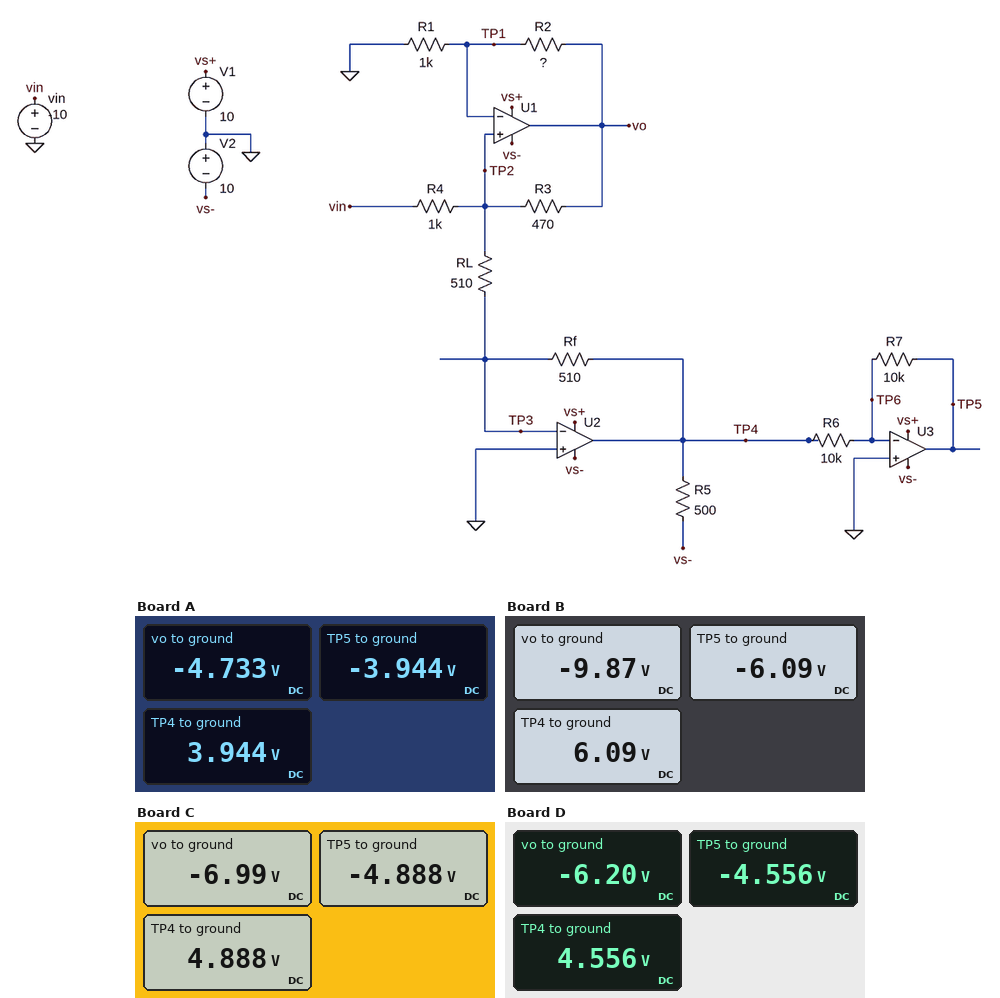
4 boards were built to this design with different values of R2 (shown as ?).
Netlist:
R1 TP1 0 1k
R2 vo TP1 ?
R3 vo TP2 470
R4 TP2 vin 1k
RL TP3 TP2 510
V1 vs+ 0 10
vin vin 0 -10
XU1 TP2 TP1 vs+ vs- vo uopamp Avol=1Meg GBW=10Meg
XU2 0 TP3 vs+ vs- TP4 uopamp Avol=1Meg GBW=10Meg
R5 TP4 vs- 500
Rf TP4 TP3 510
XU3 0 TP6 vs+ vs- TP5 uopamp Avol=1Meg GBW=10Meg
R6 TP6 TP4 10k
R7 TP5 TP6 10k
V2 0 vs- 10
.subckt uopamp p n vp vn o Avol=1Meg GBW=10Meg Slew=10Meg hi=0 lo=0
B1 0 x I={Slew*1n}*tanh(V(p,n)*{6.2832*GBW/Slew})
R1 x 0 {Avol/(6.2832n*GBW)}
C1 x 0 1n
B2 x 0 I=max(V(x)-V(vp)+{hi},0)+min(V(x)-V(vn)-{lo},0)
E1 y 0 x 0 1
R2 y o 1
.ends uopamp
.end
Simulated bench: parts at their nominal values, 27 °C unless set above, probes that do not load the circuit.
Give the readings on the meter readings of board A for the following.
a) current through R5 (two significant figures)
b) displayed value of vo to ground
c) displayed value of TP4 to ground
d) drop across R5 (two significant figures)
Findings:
28 mA
-4.733 V
3.944 V
14 V
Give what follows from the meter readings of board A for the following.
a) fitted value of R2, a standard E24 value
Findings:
200 Ω
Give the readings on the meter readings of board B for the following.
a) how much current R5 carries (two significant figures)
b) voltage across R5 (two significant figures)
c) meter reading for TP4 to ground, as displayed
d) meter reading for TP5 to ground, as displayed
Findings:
32 mA
16 V
6.09 V
-6.09 V
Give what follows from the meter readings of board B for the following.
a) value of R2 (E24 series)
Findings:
620 Ω
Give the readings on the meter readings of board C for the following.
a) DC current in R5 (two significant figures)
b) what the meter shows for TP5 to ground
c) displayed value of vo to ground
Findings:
30 mA
-4.888 V
-6.99 V
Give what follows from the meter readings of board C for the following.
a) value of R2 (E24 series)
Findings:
430 Ω
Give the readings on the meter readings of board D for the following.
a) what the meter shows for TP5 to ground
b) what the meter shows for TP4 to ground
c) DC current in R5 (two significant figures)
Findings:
-4.556 V
4.556 V
29 mA
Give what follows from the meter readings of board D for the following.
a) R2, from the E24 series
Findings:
360 Ω
